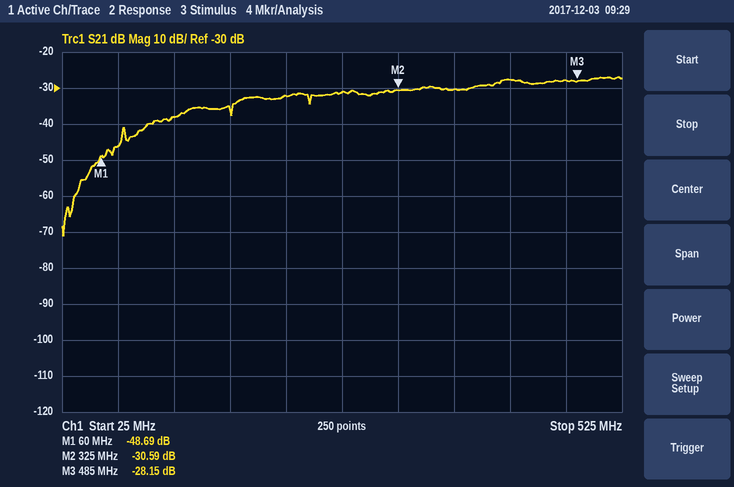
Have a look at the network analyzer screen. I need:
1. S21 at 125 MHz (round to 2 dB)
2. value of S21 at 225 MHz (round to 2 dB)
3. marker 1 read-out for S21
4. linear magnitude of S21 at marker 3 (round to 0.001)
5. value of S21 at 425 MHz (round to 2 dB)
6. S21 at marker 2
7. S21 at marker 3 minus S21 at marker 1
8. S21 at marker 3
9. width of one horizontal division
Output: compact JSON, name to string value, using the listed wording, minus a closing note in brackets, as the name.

{"S21 at 125 MHz": "-38 dB", "value of S21 at 225 MHz": "-32 dB", "marker 1 read-out for S21": "-48.69 dB", "linear magnitude of S21 at marker 3": "0.039", "value of S21 at 425 MHz": "-28 dB", "S21 at marker 2": "-30.59 dB", "S21 at marker 3 minus S21 at marker 1": "20.54 dB", "S21 at marker 3": "-28.15 dB", "width of one horizontal division": "50 MHz"}
